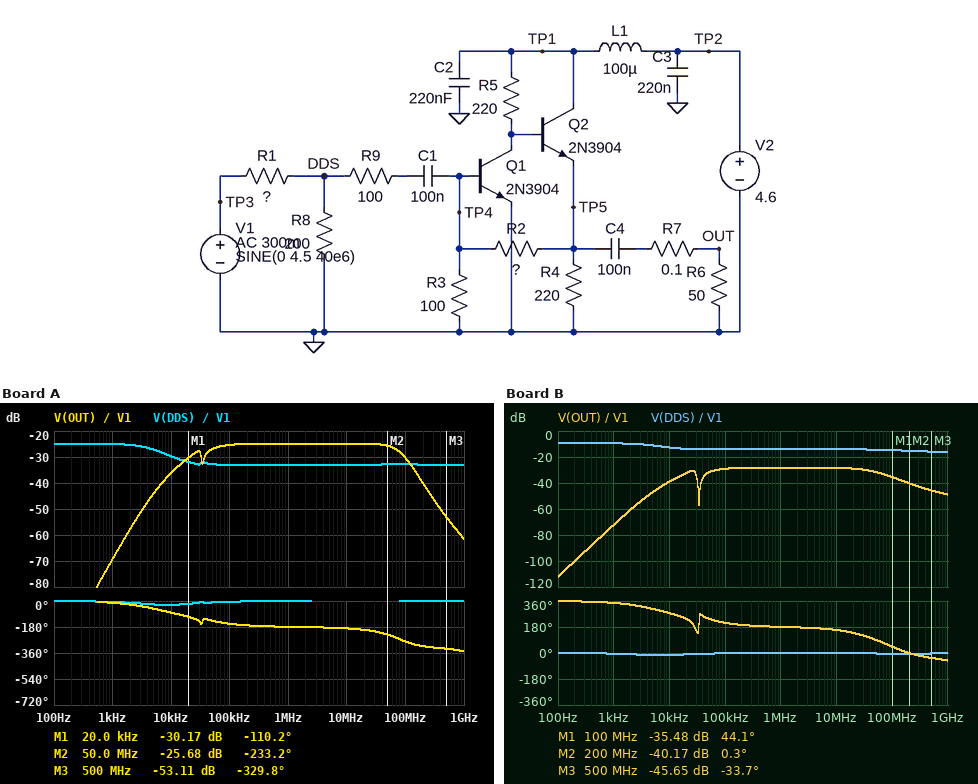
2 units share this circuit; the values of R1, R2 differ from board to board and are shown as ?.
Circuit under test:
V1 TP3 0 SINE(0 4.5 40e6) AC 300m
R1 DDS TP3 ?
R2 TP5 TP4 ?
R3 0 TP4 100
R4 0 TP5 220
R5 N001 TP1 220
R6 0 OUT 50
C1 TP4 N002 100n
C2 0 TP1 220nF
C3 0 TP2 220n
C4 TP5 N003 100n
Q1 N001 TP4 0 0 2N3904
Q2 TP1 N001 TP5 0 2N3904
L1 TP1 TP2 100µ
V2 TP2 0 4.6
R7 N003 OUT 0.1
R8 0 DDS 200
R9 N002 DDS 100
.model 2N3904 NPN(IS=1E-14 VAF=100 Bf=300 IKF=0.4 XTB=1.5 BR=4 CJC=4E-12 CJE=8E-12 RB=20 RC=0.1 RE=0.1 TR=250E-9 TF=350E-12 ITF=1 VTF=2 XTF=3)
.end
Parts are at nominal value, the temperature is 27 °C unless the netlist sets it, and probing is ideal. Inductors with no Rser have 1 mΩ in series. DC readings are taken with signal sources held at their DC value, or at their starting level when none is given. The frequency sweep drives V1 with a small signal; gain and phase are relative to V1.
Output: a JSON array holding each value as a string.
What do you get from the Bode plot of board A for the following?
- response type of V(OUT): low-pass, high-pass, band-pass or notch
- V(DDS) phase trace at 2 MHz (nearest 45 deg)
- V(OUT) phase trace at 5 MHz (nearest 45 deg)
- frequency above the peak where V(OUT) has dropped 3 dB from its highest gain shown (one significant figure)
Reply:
["band-pass", "0 deg", "-180 deg", "80 MHz"]
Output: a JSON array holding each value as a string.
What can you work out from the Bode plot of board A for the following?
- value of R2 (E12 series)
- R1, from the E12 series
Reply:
["390 Ω", "3.3 kΩ"]
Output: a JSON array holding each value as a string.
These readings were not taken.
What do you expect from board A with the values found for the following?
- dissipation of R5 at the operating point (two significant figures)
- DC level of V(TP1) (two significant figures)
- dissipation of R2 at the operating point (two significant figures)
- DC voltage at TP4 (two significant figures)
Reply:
["1.3 mW", "4.6 V", "18 mW", "680 mV"]
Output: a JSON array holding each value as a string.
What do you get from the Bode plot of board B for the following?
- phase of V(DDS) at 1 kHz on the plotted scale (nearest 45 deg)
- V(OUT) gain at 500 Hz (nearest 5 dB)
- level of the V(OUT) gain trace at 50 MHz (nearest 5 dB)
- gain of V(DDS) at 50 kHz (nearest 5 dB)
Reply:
["0 deg", "-85 dB", "-30 dB", "-15 dB"]
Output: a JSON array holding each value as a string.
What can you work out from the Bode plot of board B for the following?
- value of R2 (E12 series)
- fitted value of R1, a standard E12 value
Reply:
["560 Ω", "390 Ω"]
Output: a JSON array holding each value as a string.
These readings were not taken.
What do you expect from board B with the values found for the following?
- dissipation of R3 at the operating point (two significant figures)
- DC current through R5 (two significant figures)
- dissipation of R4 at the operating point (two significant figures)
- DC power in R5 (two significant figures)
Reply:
["3.4 mW", "140 µA", "67 mW", "4.2 µW"]
